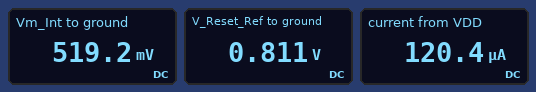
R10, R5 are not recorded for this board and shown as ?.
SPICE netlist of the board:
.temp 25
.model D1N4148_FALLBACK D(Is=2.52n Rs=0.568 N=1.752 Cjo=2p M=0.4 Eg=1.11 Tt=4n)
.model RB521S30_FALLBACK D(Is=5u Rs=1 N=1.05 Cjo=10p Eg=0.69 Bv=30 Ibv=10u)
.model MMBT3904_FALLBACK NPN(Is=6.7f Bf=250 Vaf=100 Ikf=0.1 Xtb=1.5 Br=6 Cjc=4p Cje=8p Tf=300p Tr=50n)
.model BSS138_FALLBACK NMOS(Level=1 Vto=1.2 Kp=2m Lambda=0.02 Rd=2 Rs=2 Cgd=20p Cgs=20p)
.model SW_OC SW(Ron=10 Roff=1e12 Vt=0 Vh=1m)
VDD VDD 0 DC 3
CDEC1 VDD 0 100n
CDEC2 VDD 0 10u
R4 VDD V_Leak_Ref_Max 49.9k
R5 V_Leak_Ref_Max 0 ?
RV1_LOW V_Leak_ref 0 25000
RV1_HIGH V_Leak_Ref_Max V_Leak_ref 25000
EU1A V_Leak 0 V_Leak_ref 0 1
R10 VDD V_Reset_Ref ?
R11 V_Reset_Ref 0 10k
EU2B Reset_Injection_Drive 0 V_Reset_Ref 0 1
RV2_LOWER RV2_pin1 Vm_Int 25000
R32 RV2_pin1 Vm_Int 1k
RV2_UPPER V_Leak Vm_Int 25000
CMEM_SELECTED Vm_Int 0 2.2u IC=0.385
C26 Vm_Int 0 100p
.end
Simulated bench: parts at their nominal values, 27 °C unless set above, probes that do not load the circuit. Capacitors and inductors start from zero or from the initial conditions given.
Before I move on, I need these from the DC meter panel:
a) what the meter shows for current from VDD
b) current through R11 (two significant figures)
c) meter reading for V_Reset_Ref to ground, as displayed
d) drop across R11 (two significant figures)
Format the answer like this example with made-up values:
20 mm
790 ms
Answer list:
120.4 µA
81 µA
0.811 V
810 mV
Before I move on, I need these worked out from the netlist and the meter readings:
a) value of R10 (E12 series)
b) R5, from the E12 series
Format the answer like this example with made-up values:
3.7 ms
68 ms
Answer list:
27 kΩ
56 kΩ
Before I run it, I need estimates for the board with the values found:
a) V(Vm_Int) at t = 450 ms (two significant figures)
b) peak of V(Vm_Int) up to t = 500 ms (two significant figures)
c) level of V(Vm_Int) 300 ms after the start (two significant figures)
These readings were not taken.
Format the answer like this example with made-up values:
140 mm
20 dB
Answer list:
520 mV
520 mV
520 mV
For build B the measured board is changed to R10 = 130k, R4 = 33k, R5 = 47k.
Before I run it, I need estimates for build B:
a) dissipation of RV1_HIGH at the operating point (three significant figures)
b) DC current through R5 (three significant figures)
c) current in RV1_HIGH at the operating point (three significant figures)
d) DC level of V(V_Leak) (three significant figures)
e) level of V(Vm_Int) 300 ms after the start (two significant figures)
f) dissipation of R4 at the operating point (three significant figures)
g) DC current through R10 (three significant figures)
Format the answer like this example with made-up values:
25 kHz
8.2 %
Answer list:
16.1 µW
27.0 µA
25.4 µA
635 mV
630 mV
90.7 µW
21.4 µA
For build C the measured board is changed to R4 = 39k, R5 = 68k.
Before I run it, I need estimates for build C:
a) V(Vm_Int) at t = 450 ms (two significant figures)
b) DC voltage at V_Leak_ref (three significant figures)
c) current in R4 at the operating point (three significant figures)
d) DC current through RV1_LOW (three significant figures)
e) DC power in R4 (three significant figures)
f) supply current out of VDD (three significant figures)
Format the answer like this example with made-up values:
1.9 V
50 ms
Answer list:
640 mV
637 mV
44.2 µA
25.5 µA
76.3 µW
125 µA
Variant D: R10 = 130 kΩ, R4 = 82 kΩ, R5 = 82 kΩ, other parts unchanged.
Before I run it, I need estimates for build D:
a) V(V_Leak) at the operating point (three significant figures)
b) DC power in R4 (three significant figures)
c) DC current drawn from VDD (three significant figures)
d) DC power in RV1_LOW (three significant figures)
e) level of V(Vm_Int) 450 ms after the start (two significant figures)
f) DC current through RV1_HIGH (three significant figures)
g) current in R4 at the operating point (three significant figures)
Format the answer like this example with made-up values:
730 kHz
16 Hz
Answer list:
412 mV
57.7 µW
48.0 µA
6.79 µW
410 mV
16.5 µA
26.5 µA
